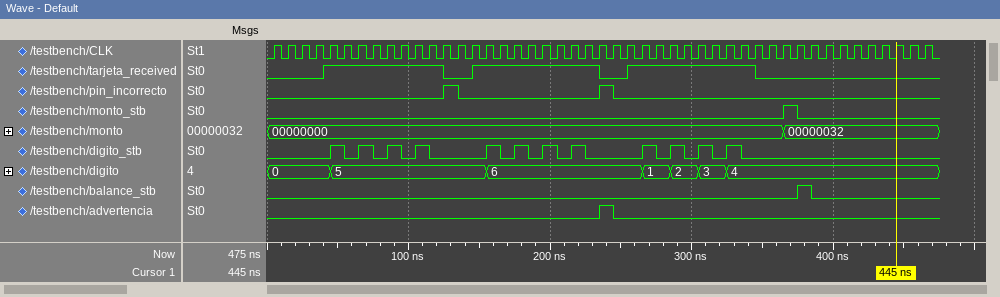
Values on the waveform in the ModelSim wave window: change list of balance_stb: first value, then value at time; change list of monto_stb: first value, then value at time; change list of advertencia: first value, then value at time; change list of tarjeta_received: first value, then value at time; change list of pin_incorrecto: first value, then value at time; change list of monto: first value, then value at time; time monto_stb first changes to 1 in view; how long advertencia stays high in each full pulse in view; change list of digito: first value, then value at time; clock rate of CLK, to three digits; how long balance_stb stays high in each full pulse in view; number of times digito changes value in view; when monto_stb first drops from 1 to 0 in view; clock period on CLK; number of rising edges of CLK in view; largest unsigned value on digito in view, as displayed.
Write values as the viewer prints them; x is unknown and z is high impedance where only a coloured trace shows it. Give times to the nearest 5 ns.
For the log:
0, 1 at 375 ns, 0 at 385 ns
0, 1 at 365 ns, 0 at 375 ns
0, 1 at 235 ns, 0 at 245 ns
0, 1 at 40 ns, 0 at 125 ns, 1 at 145 ns, 0 at 235 ns, 1 at 255 ns, 0 at 345 ns
0, 1 at 125 ns, 0 at 135 ns, 1 at 235 ns, 0 at 245 ns
00000000, 00000032 at 365 ns
365 ns
10 ns
0, 5 at 45 ns, 6 at 155 ns, 1 at 265 ns, 2 at 285 ns, 3 at 305 ns, 4 at 325 ns
100 MHz
10 ns
6
375 ns
10 ns
47
6
